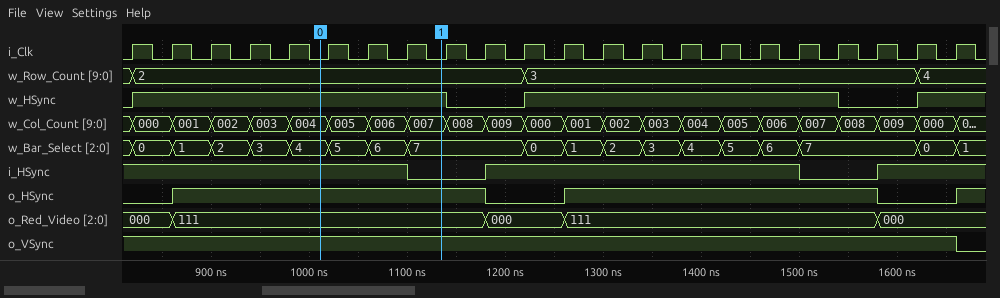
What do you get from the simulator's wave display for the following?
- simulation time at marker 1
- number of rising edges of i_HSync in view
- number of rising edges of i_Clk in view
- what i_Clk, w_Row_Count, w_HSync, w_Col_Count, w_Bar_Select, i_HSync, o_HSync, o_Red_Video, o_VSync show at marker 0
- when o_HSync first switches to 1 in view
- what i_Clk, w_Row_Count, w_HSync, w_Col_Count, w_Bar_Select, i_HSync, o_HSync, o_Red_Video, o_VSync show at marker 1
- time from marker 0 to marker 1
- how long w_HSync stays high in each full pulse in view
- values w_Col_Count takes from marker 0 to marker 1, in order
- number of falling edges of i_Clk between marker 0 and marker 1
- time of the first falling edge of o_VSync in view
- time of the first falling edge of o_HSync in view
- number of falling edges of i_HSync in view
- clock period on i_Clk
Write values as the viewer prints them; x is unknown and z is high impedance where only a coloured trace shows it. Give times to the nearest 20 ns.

1140 ns
2
22
i_Clk=0, w_Row_Count=2, w_HSync=1, w_Col_Count=004, w_Bar_Select=4, i_HSync=1, o_HSync=1, o_Red_Video=111, o_VSync=1
860 ns
i_Clk=0, w_Row_Count=2, w_HSync=1, w_Col_Count=007, w_Bar_Select=7, i_HSync=0, o_HSync=1, o_Red_Video=111, o_VSync=1
120 ns
320 ns, 320 ns
004, 005, 006, 007
3
1660 ns
1180 ns
2
40 ns
